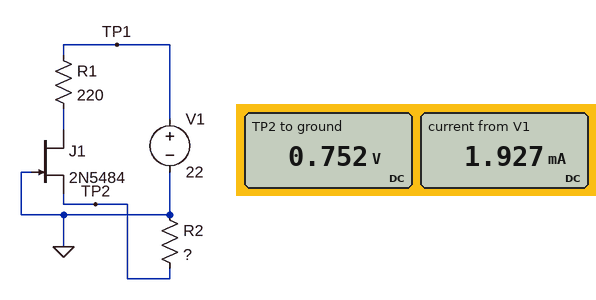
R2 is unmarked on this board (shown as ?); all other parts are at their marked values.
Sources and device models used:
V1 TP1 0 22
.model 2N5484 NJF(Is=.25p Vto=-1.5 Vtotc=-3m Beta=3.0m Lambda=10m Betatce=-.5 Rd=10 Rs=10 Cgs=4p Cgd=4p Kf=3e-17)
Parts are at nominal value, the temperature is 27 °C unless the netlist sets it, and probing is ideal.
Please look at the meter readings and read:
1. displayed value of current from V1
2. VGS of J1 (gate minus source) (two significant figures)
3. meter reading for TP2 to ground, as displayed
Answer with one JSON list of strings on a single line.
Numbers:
["1.927 mA", "-750 mV", "0.752 V"]
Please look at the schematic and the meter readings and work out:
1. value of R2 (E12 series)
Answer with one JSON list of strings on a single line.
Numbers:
["390 Ω"]
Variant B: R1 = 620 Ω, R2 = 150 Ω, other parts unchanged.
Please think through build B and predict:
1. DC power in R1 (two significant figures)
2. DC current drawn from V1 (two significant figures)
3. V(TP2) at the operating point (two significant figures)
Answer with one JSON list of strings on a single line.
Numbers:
["6.9 mW", "3.3 mA", "500 mV"]
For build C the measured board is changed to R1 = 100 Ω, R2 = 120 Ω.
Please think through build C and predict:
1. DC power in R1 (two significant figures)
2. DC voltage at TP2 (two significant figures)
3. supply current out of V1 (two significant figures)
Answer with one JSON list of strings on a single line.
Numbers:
["1.4 mW", "450 mV", "3.7 mA"]
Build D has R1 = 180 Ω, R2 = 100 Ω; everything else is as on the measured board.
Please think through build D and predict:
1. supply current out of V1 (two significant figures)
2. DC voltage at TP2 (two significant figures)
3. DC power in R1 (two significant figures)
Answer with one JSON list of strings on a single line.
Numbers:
["4.0 mA", "400 mV", "2.9 mW"]
